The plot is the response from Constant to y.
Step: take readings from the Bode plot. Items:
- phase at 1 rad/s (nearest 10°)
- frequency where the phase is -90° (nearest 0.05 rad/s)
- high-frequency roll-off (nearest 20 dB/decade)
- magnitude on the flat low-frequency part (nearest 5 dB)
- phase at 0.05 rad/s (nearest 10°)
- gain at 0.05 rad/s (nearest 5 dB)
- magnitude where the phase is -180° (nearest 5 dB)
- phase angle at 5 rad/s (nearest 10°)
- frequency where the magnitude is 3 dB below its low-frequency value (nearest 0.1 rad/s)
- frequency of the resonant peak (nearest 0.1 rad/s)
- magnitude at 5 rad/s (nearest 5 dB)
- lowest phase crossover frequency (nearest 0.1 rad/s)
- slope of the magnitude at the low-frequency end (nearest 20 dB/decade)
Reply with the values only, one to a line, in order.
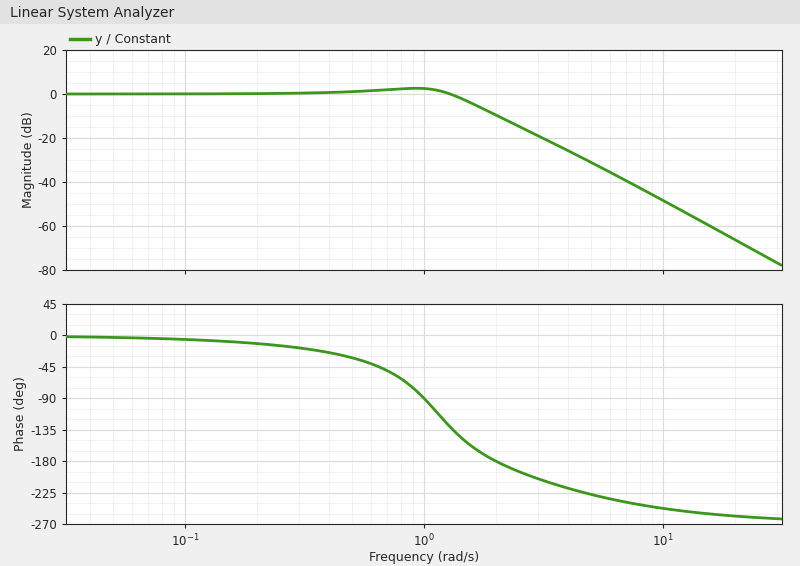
-90°
1.00 rad/s
-60 dB/decade
0 dB
0°
0 dB
-10 dB
-230°
1.5 rad/s
0.9 rad/s
-30 dB
2.0 rad/s
0 dB/decade
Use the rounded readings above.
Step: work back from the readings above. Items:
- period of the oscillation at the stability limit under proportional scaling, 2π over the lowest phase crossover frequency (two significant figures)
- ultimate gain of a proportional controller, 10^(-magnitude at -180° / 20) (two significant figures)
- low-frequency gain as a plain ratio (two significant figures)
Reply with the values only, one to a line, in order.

3.1 s
3.2
1.0
